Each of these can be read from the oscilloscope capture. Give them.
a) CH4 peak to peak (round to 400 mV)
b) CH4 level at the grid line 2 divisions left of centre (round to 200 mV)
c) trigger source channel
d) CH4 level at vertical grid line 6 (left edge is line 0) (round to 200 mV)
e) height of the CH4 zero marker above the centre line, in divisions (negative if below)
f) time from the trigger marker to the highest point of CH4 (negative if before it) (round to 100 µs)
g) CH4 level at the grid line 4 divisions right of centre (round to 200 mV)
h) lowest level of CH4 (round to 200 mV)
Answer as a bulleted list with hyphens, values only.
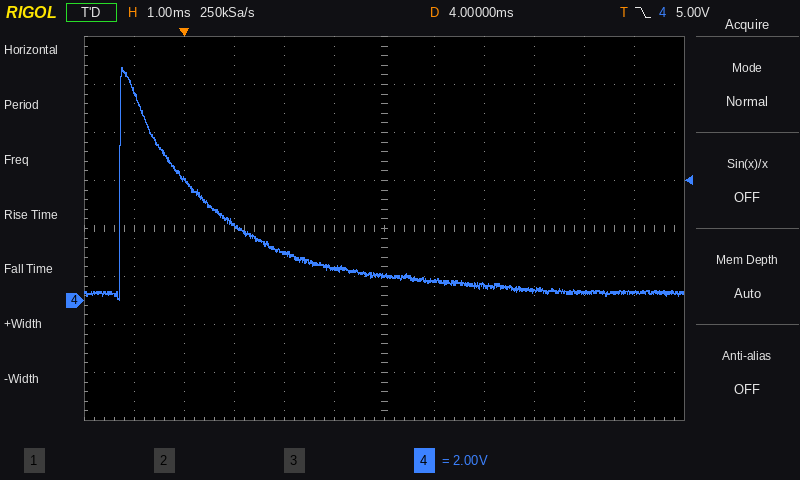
- 9.6 V
- 2.0 V
- CH4
- 1.0 V
- -1.5 div
- -1.2 ms
- 400 mV
- 0.0 V
